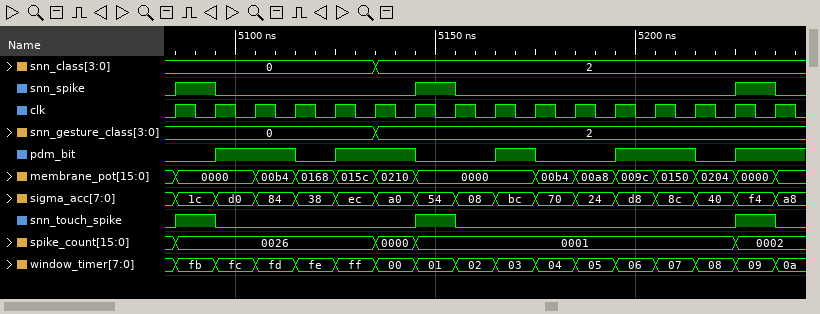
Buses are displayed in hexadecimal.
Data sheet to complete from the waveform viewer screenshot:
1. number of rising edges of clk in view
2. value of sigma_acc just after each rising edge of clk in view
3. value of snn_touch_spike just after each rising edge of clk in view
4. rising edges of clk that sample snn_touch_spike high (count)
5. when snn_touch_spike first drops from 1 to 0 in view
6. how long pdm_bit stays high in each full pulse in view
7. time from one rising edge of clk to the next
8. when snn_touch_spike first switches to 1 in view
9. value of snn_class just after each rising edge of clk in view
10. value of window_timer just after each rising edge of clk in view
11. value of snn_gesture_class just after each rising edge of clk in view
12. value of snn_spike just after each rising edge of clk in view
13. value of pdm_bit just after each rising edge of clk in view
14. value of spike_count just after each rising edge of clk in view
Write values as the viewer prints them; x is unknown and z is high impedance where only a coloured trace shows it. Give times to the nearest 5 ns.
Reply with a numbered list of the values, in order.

1. 16
2. 1c, d0, 84, 38, ec, a0, 54, 08, bc, 70, 24, d8, 8c, 40, f4, a8
3. 1 0 0 0 0 0 1 0 0 0 0 0 0 0 1 0
4. 3
5. 5095 ns
6. 20 ns, 20 ns, 10 ns, 20 ns
7. 10 ns
8. 5085 ns
9. 0, 0, 0, 0, 0, 2, 2, 2, 2, 2, 2, 2, 2, 2, 2, 2
10. fb, fc, fd, fe, ff, 00, 01, 02, 03, 04, 05, 06, 07, 08, 09, 0a
11. 0, 0, 0, 0, 0, 2, 2, 2, 2, 2, 2, 2, 2, 2, 2, 2
12. 1 0 0 0 0 0 1 0 0 0 0 0 0 0 1 0
13. 0 1 1 0 1 1 0 0 1 0 0 1 1 0 1 1
14. 0026, 0026, 0026, 0026, 0026, 0000, 0001, 0001, 0001, 0001, 0001, 0001, 0001, 0001, 0002, 0002
